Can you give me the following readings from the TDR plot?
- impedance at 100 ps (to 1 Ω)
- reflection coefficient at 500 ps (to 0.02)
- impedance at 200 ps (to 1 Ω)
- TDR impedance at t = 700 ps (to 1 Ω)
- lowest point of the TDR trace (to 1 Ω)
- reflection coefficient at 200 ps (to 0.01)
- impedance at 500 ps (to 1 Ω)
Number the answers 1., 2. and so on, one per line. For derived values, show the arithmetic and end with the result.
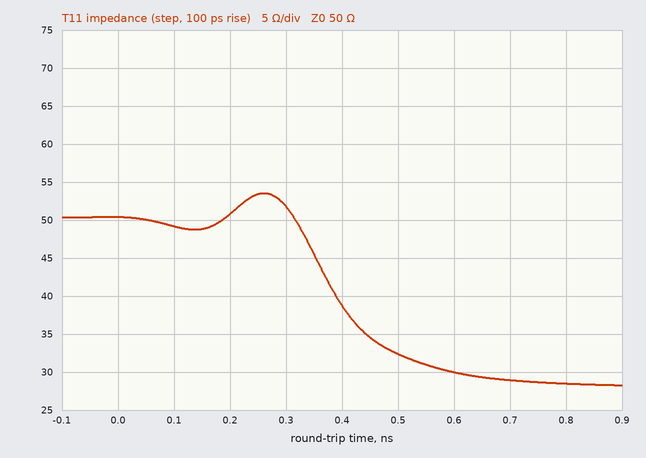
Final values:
1. 49 Ω
2. (32 − 50)/(32 + 50) ≈ -0.22
3. 51 Ω
4. 29 Ω
5. 28 Ω
6. (51 − 50)/(51 + 50) ≈ +0.01
7. 32 Ω
